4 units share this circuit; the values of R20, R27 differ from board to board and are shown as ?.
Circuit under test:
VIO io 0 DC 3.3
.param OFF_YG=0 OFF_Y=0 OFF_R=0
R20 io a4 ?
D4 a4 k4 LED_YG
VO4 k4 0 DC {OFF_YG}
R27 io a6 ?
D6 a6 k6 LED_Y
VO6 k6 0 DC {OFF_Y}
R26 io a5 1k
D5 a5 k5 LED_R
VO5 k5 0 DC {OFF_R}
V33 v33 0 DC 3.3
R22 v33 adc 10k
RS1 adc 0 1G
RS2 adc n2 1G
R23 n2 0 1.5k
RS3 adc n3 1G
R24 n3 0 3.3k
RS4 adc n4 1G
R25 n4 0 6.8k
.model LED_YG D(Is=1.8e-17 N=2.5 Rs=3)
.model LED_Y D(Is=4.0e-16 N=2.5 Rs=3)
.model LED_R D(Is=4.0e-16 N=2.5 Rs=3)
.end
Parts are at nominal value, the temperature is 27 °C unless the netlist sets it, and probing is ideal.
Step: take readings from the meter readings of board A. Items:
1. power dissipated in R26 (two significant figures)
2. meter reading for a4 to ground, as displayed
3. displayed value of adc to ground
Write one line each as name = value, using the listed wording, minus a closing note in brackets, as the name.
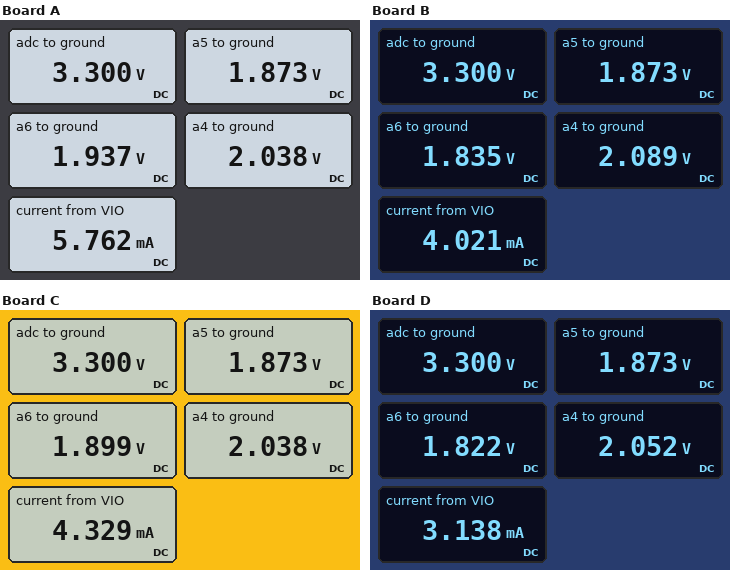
power dissipated in R26 = 2.0 mW
meter reading for a4 to ground, as displayed = 2.038 V
displayed value of adc to ground = 3.300 V
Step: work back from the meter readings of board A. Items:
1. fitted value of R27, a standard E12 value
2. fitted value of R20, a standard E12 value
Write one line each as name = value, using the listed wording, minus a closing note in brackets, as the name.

fitted value of R27, a standard E12 value = 390 Ω
fitted value of R20, a standard E12 value = 1.5 kΩ
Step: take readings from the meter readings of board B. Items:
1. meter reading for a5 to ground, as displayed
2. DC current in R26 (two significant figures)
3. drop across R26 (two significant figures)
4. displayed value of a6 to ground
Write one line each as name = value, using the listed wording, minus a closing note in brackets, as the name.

meter reading for a5 to ground, as displayed = 1.873 V
DC current in R26 = 1.4 mA
drop across R26 = 1.4 V
displayed value of a6 to ground = 1.835 V
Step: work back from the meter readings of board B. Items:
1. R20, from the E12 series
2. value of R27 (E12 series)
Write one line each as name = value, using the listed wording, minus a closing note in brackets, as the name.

R20, from the E12 series = 680 Ω
value of R27 = 1.8 kΩ
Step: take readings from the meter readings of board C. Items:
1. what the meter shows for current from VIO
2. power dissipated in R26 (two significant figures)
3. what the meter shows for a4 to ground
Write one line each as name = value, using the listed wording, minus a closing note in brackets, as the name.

what the meter shows for current from VIO = 4.329 mA
power dissipated in R26 = 2.0 mW
what the meter shows for a4 to ground = 2.038 V
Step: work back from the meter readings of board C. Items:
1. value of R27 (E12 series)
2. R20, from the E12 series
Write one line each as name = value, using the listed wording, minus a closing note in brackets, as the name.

value of R27 = 680 Ω
R20, from the E12 series = 1.5 kΩ
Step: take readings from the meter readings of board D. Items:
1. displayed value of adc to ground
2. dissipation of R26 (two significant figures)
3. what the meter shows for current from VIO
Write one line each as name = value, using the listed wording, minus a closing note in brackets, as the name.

displayed value of adc to ground = 3.300 V
dissipation of R26 = 2.0 mW
what the meter shows for current from VIO = 3.138 mA
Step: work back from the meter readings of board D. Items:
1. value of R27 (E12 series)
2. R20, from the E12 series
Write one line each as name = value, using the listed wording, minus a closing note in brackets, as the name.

value of R27 = 2.2 kΩ
R20, from the E12 series = 1.2 kΩ
